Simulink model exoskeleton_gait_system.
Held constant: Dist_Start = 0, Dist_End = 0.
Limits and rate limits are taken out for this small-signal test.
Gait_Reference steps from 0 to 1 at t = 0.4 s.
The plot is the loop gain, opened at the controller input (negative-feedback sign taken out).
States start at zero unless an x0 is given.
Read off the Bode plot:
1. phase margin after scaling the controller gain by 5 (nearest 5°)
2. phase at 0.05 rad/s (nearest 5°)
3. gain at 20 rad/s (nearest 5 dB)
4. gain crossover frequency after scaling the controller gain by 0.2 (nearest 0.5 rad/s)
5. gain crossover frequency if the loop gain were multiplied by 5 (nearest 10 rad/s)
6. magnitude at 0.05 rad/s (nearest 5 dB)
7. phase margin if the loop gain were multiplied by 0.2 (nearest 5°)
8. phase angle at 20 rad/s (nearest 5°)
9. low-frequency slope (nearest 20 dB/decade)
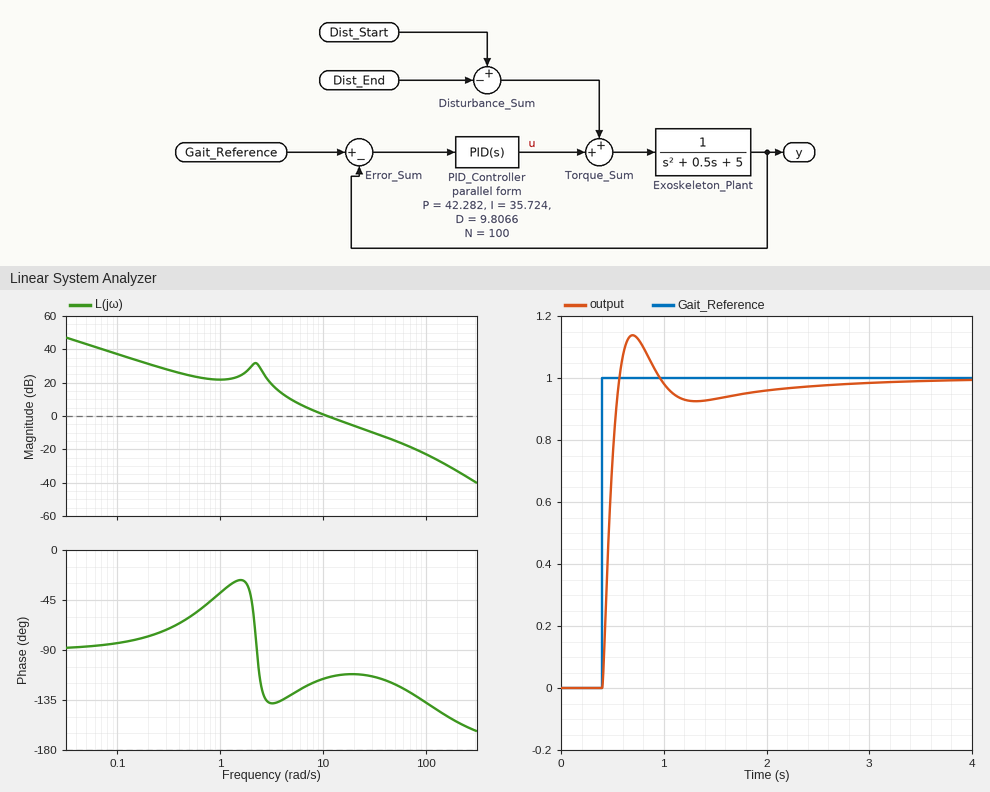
60°
-85°
-5 dB
4.0 rad/s
50 rad/s
45 dB
45°
-110°
-20 dB/decade
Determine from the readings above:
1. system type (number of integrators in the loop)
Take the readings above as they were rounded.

1
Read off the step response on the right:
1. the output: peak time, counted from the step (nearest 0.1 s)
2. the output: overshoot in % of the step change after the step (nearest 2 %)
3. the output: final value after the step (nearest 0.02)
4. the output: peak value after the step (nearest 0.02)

0.3 s
14 %
1.00
1.14
